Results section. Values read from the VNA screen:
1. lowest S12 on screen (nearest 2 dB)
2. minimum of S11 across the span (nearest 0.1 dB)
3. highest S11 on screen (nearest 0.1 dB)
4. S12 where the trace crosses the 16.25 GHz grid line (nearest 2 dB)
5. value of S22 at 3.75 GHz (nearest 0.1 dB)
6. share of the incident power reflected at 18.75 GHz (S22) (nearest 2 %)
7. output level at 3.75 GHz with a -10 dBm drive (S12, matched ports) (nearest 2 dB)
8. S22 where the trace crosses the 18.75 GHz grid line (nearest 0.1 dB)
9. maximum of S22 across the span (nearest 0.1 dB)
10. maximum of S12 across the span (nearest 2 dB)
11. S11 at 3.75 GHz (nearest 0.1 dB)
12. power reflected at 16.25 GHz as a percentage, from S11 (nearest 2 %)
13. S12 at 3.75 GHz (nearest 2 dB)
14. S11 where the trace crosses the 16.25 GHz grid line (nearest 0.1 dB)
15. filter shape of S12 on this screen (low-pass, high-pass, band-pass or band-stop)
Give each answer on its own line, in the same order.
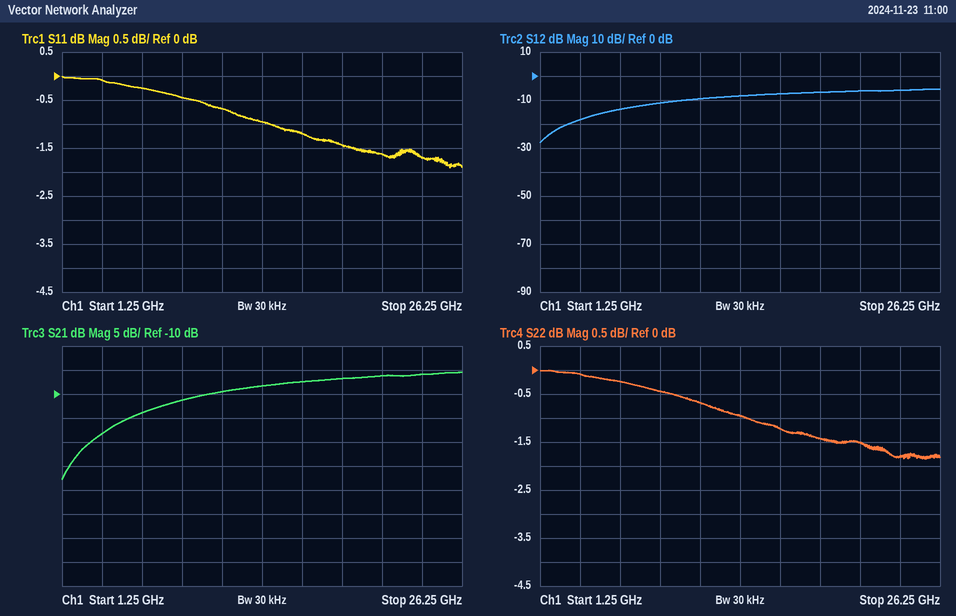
-28 dB
-1.9 dB
0.0 dB
-8 dB
-0.1 dB
72 %
-28 dBm
-1.4 dB
0.0 dB
-6 dB
-0.1 dB
76 %
-18 dB
-1.2 dB
high-pass
